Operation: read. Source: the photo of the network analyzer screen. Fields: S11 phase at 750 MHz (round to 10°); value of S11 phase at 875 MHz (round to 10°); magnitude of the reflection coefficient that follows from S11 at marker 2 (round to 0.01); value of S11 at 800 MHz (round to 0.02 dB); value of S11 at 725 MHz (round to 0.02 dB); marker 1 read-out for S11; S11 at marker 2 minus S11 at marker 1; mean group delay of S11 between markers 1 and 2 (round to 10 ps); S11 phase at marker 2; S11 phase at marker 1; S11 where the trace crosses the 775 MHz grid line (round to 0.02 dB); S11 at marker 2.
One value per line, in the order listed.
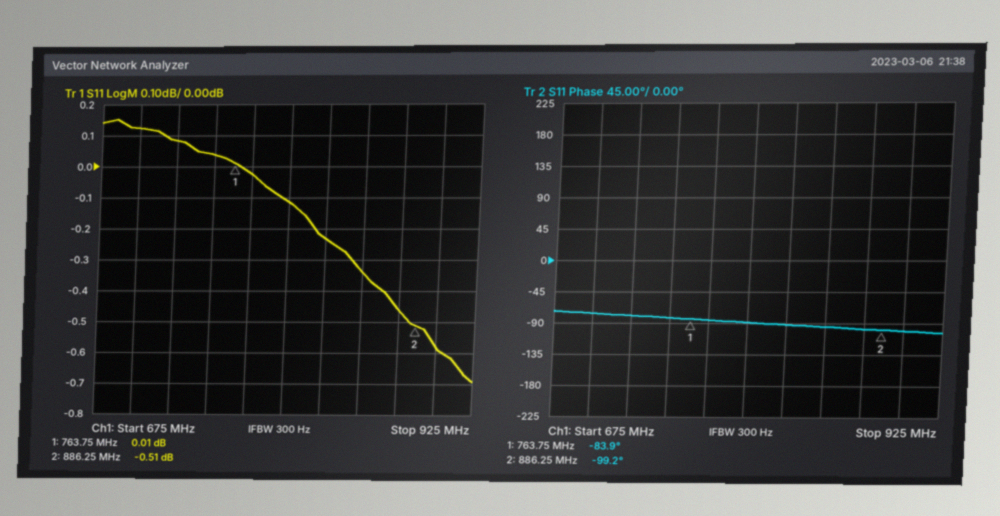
-80°
-100°
0.94
-0.12 dB
0.08 dB
0.01 dB
-0.52 dB
350 ps
-99.2°
-83.9°
-0.02 dB
-0.51 dB
